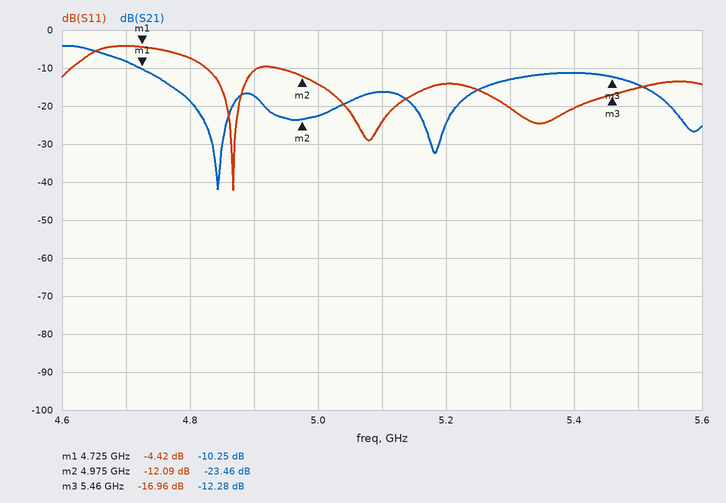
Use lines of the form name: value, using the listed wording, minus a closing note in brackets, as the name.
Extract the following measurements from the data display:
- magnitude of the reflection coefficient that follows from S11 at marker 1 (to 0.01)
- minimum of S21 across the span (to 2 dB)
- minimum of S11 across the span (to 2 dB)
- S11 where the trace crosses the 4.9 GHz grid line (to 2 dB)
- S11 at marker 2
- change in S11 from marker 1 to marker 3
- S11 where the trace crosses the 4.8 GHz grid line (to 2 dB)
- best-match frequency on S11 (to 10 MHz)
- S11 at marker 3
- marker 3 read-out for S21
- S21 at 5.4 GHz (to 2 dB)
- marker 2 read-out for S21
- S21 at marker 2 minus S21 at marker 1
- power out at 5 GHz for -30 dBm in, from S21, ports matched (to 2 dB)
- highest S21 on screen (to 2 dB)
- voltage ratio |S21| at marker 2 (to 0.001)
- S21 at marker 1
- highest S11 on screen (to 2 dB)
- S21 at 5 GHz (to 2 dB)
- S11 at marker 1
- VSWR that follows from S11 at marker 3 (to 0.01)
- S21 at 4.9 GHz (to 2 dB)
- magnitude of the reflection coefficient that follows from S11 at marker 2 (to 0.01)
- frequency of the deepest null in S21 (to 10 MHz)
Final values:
magnitude of the reflection coefficient that follows from S11 at marker 1: 0.60
minimum of S21 across the span: -42 dB
minimum of S11 across the span: -42 dB
S11 where the trace crosses the 4.9 GHz grid line: -10 dB
S11 at marker 2: -12.09 dB
change in S11 from marker 1 to marker 3: -12.54 dB
S11 where the trace crosses the 4.8 GHz grid line: -8 dB
best-match frequency on S11: 4.87 GHz
S11 at marker 3: -16.96 dB
marker 3 read-out for S21: -12.28 dB
S21 at 5.4 GHz: -12 dB
marker 2 read-out for S21: -23.46 dB
S21 at marker 2 minus S21 at marker 1: -13.21 dB
power out at 5 GHz for -30 dBm in, from S21, ports matched: -52 dBm
highest S21 on screen: -4 dB
voltage ratio |S21| at marker 2: 0.067
S21 at marker 1: -10.25 dB
highest S11 on screen: -4 dB
S21 at 5 GHz: -22 dB
S11 at marker 1: -4.42 dB
VSWR that follows from S11 at marker 3: 1.33
S21 at 4.9 GHz: -18 dB
magnitude of the reflection coefficient that follows from S11 at marker 2: 0.25
frequency of the deepest null in S21: 4.84 GHz
